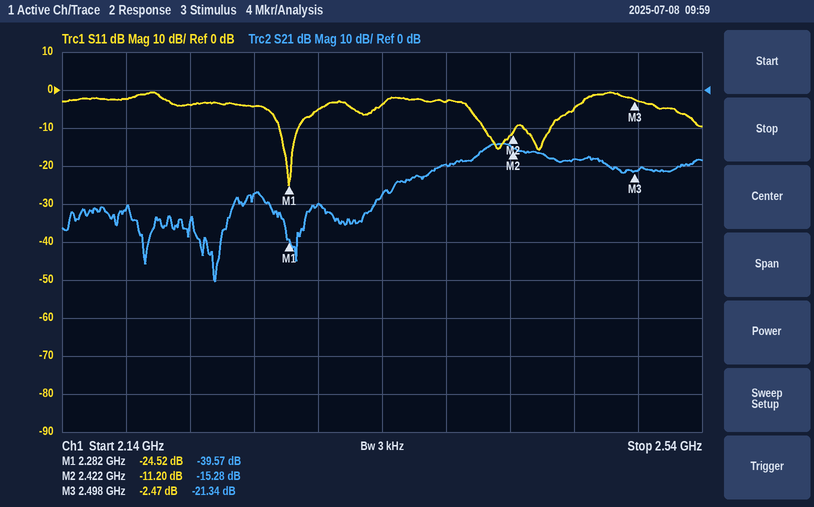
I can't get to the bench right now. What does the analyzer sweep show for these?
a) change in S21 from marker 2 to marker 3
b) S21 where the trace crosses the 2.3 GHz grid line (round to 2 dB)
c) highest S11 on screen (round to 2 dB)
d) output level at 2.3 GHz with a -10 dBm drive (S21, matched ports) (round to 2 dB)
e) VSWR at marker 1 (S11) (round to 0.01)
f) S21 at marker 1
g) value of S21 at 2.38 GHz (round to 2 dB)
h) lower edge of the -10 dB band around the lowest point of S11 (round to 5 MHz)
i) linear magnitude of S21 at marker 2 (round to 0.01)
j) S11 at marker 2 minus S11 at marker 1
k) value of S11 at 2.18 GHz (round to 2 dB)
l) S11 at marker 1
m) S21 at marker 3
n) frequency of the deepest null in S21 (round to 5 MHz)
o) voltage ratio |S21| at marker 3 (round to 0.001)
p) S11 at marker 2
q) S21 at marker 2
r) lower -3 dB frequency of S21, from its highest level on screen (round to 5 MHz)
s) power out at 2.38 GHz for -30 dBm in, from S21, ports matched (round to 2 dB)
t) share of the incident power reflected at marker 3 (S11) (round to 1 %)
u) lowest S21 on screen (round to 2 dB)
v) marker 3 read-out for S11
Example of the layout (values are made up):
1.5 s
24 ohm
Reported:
-6.06 dB
-30 dB
0 dB
-40 dBm
1.13
-39.57 dB
-20 dB
2.275 GHz
0.17
13.32 dB
-2 dB
-24.52 dB
-21.34 dB
2.235 GHz
0.086
-11.20 dB
-15.28 dB
2.400 GHz
-50 dBm
57 %
-50 dB
-2.47 dB
